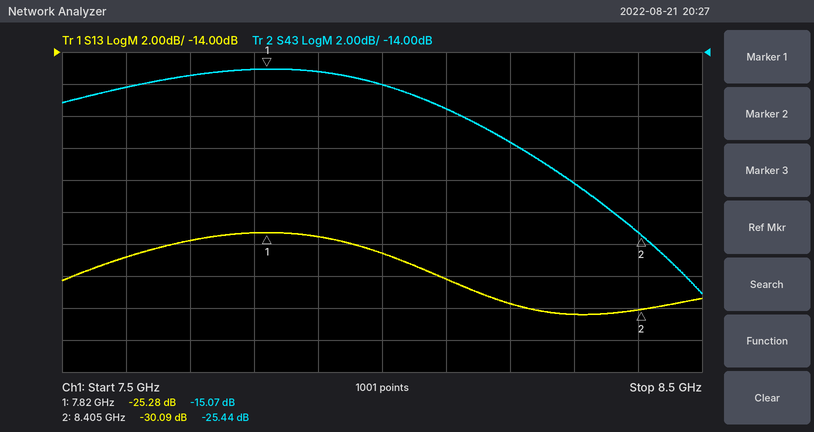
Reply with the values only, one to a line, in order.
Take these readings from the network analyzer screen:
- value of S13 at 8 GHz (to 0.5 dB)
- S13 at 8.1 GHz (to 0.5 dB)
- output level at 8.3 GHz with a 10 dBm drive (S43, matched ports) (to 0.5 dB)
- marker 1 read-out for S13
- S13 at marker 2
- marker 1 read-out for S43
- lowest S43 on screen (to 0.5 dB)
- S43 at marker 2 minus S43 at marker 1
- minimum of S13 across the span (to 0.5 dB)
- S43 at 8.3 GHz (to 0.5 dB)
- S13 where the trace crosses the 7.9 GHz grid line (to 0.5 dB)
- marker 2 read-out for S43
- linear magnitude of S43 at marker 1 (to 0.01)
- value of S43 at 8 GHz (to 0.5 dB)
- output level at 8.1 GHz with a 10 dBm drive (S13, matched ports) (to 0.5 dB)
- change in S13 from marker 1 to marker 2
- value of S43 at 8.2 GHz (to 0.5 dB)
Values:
-26.5 dB
-28.0 dB
-12.0 dBm
-25.28 dB
-30.09 dB
-15.07 dB
-29.0 dB
-10.37 dB
-30.5 dB
-22.0 dB
-25.5 dB
-25.44 dB
0.18
-16.0 dB
-18.0 dBm
-4.81 dB
-19.5 dB
